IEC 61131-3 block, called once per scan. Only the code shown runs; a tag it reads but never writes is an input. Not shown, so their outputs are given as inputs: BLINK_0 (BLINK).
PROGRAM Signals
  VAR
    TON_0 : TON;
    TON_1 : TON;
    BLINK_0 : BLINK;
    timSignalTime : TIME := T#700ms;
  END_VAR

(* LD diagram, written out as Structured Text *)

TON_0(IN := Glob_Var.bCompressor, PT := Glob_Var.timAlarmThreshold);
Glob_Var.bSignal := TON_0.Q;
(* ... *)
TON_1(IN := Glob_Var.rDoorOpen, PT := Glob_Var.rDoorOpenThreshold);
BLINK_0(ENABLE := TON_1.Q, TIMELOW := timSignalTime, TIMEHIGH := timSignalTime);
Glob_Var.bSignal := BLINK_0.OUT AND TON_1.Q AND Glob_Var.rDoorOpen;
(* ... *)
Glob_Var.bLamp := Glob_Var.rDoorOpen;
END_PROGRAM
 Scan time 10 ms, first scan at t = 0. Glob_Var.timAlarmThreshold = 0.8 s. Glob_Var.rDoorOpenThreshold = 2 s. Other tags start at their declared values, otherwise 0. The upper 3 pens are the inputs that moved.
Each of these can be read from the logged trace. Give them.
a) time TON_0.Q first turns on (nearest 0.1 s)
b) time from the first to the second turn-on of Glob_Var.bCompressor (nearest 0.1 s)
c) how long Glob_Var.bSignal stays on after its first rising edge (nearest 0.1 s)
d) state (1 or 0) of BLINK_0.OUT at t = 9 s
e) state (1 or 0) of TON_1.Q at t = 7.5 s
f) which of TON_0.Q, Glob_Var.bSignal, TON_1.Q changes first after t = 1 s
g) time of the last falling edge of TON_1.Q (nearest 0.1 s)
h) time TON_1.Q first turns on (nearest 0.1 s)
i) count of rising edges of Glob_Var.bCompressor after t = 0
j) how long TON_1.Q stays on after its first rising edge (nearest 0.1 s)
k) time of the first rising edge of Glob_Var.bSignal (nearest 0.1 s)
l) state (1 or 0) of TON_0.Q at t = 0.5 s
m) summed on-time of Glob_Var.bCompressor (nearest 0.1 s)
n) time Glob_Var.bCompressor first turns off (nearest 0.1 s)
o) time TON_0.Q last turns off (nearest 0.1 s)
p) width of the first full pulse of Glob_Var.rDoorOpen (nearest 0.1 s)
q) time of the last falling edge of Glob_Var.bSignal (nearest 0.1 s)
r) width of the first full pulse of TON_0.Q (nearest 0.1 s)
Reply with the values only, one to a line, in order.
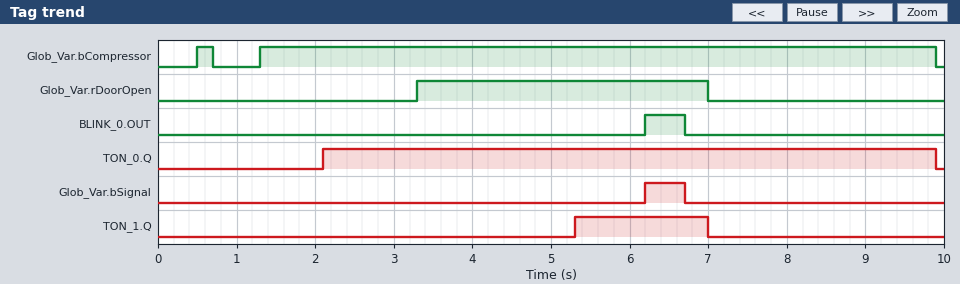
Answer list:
2.1 s
0.8 s
0.5 s
0
0
TON_0.Q
7.0 s
5.3 s
2
1.7 s
6.2 s
0
8.8 s
0.7 s
9.9 s
3.7 s
6.7 s
7.8 s
